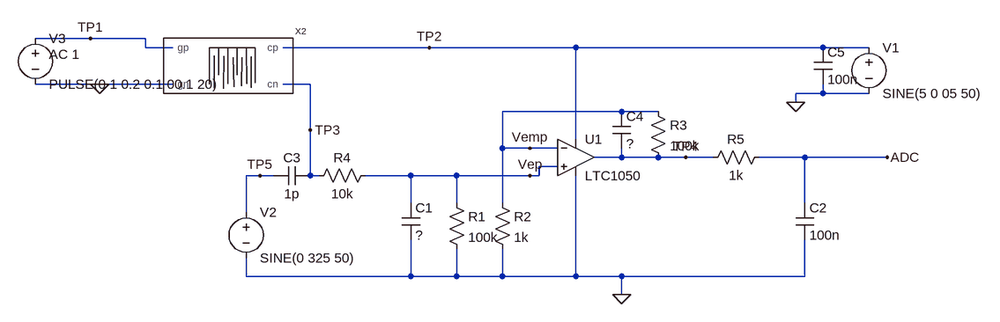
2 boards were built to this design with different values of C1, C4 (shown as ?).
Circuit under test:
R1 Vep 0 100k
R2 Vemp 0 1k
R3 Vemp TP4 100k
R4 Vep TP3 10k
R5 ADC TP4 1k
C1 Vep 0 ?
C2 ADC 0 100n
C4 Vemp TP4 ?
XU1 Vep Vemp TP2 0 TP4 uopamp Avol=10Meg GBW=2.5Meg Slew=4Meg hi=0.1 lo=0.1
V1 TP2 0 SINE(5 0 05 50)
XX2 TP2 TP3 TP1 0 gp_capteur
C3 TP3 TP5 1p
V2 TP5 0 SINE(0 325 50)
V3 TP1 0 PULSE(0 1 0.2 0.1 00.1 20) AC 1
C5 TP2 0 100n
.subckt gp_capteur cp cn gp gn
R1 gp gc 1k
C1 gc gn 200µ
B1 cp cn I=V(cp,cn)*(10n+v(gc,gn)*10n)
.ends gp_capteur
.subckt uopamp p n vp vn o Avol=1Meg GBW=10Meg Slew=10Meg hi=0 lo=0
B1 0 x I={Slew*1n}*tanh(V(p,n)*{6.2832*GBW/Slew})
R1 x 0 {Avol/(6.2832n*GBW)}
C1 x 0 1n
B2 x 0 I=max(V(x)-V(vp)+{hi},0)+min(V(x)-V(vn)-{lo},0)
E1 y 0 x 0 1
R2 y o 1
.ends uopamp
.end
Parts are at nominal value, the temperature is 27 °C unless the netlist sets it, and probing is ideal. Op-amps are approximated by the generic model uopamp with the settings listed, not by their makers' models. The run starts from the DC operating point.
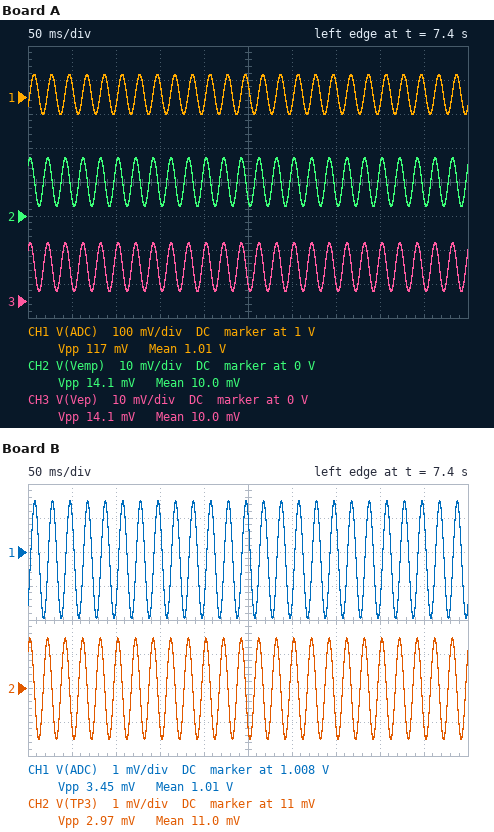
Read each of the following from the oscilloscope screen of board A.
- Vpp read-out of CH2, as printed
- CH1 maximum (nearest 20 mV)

14.1 mV
1.06 V
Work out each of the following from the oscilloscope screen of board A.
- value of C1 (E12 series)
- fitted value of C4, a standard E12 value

33 nF
390 nF
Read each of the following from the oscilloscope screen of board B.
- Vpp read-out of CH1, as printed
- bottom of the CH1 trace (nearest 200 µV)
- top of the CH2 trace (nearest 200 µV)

3.45 mV
1.0060 V
12.4 mV
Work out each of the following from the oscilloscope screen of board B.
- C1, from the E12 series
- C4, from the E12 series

330 nF
2.2 µF
